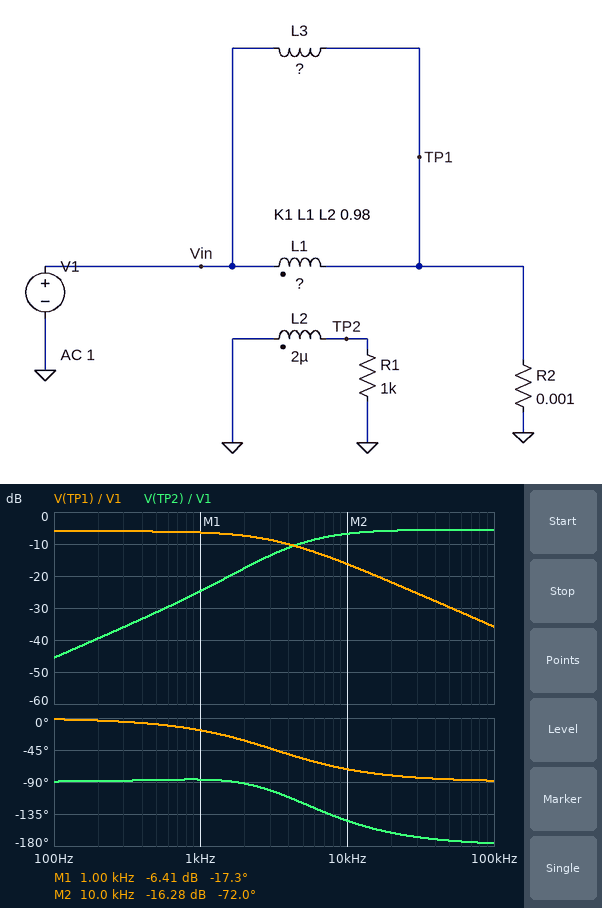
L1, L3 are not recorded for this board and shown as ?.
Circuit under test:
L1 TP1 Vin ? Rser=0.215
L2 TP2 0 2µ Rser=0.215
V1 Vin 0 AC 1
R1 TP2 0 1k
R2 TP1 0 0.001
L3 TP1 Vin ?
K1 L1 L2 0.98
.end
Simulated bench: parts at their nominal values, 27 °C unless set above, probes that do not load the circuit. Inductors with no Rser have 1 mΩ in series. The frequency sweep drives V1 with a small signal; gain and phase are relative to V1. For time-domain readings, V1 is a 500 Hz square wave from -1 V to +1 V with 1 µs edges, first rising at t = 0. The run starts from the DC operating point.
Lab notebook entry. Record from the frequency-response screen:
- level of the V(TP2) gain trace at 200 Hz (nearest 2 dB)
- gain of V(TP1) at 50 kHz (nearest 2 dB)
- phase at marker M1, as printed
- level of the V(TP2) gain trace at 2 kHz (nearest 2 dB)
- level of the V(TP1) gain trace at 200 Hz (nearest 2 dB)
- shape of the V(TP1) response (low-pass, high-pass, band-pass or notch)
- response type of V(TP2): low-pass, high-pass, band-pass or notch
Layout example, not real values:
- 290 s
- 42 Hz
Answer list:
- -40 dB
- -30 dB
- -17.3 deg
- -18 dB
- -6 dB
- low-pass
- high-pass
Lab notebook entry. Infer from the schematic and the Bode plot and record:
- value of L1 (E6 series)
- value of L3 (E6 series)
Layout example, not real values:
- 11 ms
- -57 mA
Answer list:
- 6.8 µH
- 100 nH
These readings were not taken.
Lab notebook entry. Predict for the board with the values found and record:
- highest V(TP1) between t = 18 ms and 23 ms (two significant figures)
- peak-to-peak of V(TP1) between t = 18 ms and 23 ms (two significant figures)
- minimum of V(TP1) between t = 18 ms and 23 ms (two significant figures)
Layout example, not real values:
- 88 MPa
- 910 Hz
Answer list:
- 500 mV
- 1.0 V
- -500 mV
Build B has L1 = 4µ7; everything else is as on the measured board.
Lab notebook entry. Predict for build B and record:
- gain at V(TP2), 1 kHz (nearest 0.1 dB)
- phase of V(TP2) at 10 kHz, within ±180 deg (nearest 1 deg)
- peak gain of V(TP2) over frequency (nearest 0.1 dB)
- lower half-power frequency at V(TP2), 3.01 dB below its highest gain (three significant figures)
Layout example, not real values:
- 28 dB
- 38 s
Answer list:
- -26.2 dB
- -135 deg
- -3.9 dB
- 8.17 kHz
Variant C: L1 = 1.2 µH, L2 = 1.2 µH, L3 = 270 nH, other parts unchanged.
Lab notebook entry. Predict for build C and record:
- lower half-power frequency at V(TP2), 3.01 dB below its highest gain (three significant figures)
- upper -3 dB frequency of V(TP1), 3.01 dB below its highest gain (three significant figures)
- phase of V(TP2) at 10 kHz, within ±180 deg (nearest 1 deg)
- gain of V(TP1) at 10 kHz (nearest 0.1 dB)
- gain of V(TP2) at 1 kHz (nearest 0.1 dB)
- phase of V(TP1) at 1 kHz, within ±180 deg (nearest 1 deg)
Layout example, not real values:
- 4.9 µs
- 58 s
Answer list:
- 28.7 kHz
- 1.18 kHz
- -106 deg
- -24.4 dB
- -31.8 dB
- -40 deg
